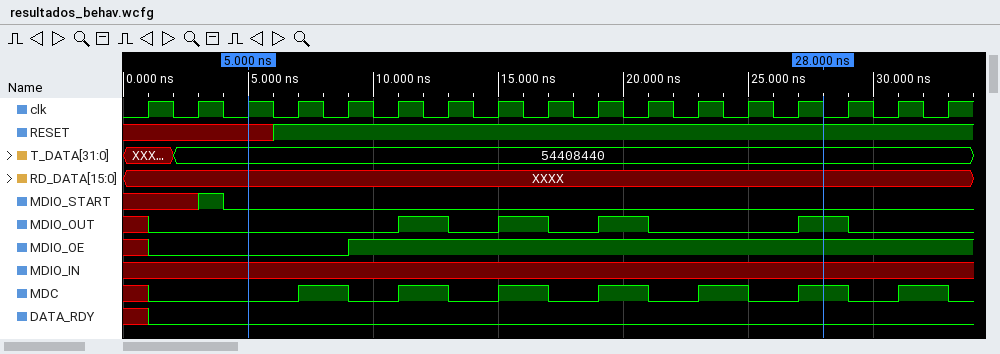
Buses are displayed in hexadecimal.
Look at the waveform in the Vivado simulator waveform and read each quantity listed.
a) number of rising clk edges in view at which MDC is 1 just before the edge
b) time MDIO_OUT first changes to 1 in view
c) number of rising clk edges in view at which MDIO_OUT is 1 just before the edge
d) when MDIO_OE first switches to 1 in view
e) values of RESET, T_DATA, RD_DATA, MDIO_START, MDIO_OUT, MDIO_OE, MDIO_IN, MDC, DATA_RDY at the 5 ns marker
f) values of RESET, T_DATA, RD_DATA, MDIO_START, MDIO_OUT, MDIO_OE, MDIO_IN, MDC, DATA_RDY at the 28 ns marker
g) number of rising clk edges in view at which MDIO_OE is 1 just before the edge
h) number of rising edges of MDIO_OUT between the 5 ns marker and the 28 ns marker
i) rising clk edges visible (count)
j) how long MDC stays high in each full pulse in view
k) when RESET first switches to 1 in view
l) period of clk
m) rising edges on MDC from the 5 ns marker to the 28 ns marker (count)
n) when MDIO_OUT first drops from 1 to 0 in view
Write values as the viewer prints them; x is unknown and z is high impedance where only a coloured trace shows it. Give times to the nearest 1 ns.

7
11 ns
4
9 ns
RESET=x, T_DATA=54408440, RD_DATA=XXXX, MDIO_START=0, MDIO_OUT=0, MDIO_OE=0, MDIO_IN=x, MDC=0, DATA_RDY=0
RESET=1, T_DATA=54408440, RD_DATA=XXXX, MDIO_START=0, MDIO_OUT=1, MDIO_OE=1, MDIO_IN=x, MDC=1, DATA_RDY=0
12
4
17
2 ns, 2 ns, 2 ns, 2 ns, 2 ns, 2 ns, 2 ns
6 ns
2 ns
6
13 ns
